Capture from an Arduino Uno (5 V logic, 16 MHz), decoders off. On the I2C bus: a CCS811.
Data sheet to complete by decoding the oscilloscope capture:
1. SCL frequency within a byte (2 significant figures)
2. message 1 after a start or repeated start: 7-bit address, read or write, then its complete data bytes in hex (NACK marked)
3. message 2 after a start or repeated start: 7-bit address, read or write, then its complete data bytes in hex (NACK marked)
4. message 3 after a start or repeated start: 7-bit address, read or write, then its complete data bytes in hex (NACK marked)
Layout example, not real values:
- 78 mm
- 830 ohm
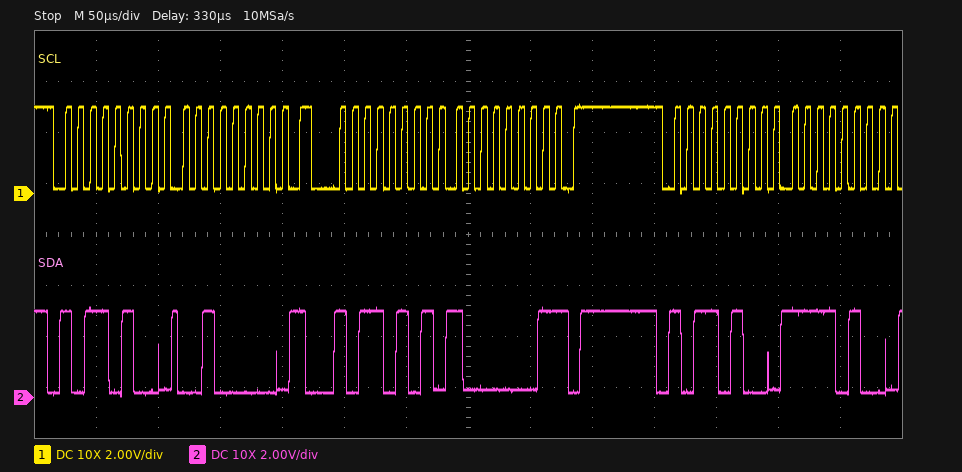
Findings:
- 100 kHz
- 0x5A write: 20
- 0x5A read: 81 NACK
- 0x5A write: F4
